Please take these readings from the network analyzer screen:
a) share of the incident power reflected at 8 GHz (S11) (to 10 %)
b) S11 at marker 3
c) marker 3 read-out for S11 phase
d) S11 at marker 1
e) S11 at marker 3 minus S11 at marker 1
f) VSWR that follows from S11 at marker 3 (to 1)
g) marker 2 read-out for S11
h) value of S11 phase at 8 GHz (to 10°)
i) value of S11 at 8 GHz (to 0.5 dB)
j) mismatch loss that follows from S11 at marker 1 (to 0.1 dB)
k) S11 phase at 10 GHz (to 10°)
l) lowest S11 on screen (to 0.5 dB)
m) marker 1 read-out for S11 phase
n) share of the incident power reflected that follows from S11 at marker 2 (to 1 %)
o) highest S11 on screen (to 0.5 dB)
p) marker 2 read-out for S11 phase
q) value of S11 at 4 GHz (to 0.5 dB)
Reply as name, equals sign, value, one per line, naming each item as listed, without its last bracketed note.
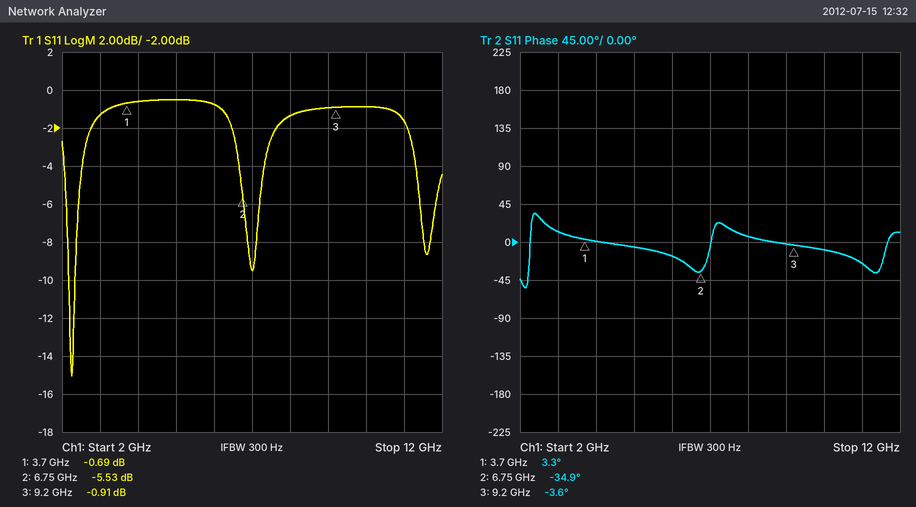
share of the incident power reflected at 8 GHz (S11) = 70 %
S11 at marker 3 = -0.91 dB
marker 3 read-out for S11 phase = -3.6°
S11 at marker 1 = -0.69 dB
S11 at marker 3 minus S11 at marker 1 = -0.22 dB
VSWR that follows from S11 at marker 3 = 19
marker 2 read-out for S11 = -5.53 dB
value of S11 phase at 8 GHz = 10°
value of S11 at 8 GHz = -1.5 dB
mismatch loss that follows from S11 at marker 1 = 8.3 dB
S11 phase at 10 GHz = -10°
lowest S11 on screen = -15.0 dB
marker 1 read-out for S11 phase = 3.3°
share of the incident power reflected that follows from S11 at marker 2 = 28 %
highest S11 on screen = -0.5 dB
marker 2 read-out for S11 phase = -34.9°
value of S11 at 4 GHz = -0.5 dB
